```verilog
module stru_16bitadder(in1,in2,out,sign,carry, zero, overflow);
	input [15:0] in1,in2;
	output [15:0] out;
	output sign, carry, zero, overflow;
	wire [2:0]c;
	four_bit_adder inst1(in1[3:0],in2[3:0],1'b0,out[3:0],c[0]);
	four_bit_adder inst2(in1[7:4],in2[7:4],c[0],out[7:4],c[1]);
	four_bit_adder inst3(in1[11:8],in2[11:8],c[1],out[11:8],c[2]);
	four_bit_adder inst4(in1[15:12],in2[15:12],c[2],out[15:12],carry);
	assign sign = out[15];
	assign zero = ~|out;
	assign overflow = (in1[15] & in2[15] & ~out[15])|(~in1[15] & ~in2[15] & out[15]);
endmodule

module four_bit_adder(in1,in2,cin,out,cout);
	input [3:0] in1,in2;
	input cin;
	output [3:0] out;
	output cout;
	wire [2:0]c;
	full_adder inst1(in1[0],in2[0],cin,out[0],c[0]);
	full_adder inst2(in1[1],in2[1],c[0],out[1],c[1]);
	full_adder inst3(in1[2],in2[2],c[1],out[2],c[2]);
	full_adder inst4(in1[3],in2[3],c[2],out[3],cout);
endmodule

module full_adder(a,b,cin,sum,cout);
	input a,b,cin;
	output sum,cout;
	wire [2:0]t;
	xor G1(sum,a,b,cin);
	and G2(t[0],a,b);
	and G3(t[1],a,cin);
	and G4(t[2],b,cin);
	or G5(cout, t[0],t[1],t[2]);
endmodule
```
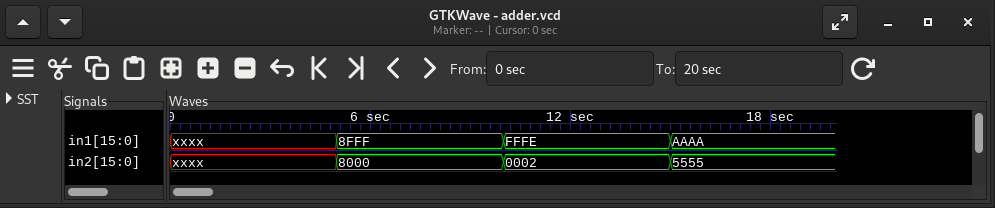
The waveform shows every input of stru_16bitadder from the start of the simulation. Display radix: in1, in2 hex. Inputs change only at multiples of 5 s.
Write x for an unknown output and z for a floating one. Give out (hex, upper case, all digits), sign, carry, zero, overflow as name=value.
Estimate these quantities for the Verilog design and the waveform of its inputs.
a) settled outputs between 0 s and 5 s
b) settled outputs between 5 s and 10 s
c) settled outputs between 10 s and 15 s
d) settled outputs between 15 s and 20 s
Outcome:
out=x, sign=x, carry=x, zero=x, overflow=x
out=0FFF, sign=0, carry=1, zero=0, overflow=1
out=0000, sign=0, carry=1, zero=1, overflow=0
out=FFFF, sign=1, carry=0, zero=0, overflow=0
